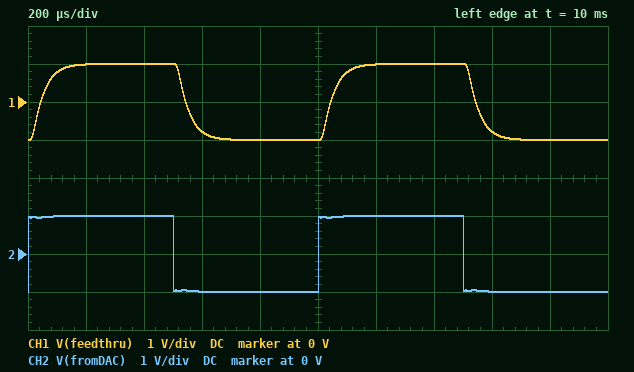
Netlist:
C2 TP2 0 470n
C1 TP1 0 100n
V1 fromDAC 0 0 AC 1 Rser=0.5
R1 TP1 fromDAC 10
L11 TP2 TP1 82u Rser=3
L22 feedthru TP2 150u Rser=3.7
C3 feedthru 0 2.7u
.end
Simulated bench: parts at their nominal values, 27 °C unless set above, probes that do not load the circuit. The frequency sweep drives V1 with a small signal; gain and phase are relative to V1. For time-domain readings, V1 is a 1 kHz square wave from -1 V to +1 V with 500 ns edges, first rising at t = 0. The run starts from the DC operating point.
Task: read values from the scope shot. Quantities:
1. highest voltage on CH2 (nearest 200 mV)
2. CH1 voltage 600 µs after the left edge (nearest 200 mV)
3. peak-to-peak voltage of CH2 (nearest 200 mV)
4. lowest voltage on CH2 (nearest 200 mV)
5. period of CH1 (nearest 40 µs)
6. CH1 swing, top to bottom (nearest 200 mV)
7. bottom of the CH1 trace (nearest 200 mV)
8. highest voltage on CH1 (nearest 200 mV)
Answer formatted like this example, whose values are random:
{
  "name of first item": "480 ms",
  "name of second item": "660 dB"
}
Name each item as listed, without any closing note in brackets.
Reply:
{
  "highest voltage on CH2": "1.0 V",
  "CH1 voltage 600 µs after the left edge": "-800 mV",
  "peak-to-peak voltage of CH2": "2.0 V",
  "lowest voltage on CH2": "-1.0 V",
  "period of CH1": "1.00 ms",
  "CH1 swing, top to bottom": "2.0 V",
  "bottom of the CH1 trace": "-1.0 V",
  "highest voltage on CH1": "1.0 V"
}
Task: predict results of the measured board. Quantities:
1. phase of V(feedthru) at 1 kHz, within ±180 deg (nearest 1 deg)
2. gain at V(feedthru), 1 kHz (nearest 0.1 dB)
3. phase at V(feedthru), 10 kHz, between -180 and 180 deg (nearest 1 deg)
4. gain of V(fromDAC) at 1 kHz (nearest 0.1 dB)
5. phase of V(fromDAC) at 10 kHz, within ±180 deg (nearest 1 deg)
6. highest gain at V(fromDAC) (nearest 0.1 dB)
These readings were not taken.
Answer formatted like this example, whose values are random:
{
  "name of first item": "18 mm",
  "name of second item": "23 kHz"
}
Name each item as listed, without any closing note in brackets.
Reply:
{
  "phase of V(feedthru) at 1 kHz, within ±180 deg": "-19 deg",
  "gain at V(feedthru), 1 kHz": "-0.2 dB",
  "phase at V(feedthru), 10 kHz, between -180 and 180 deg": "-124 deg",
  "gain of V(fromDAC) at 1 kHz": "0 dB",
  "phase of V(fromDAC) at 10 kHz, within ±180 deg": "1 deg",
  "highest gain at V(fromDAC)": "0 dB"
}
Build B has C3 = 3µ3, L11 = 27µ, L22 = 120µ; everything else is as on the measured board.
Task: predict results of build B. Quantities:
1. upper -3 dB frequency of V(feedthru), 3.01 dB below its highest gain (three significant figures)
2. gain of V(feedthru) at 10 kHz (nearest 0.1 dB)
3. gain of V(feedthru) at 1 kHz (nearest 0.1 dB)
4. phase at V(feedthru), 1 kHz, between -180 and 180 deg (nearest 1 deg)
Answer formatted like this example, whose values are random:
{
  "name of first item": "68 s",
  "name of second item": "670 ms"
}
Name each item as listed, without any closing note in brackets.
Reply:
{
  "upper -3 dB frequency of V(feedthru), 3.01 dB below its highest gain": "2.95 kHz",
  "gain of V(feedthru) at 10 kHz": "-10.8 dB",
  "gain of V(feedthru) at 1 kHz": "-0.5 dB",
  "phase at V(feedthru), 1 kHz, between -180 and 180 deg": "-22 deg"
}
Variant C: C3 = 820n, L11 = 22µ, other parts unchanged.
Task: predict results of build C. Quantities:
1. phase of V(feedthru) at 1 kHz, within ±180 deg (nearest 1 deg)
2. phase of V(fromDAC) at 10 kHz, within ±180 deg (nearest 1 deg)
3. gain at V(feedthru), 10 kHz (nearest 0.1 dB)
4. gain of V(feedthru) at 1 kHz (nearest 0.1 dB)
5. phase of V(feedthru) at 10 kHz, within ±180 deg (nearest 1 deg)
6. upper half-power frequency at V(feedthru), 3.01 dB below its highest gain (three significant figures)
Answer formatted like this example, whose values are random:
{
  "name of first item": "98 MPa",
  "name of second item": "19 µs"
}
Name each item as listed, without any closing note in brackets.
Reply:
{
  "phase of V(feedthru) at 1 kHz, within ±180 deg": "-8 deg",
  "phase of V(fromDAC) at 10 kHz, within ±180 deg": "-1 deg",
  "gain at V(feedthru), 10 kHz": "-1.3 dB",
  "gain of V(feedthru) at 1 kHz": "0 dB",
  "phase of V(feedthru) at 10 kHz, within ±180 deg": "-74 deg",
  "upper half-power frequency at V(feedthru), 3.01 dB below its highest gain": "17.2 kHz"
}
